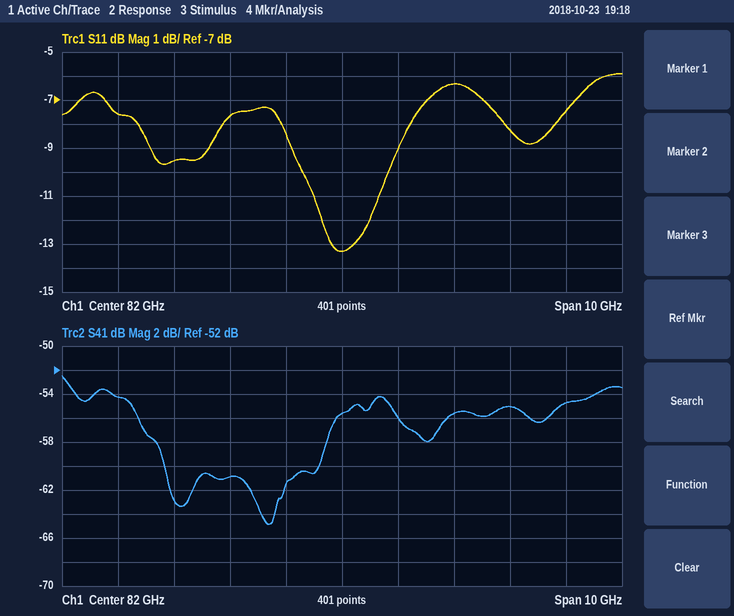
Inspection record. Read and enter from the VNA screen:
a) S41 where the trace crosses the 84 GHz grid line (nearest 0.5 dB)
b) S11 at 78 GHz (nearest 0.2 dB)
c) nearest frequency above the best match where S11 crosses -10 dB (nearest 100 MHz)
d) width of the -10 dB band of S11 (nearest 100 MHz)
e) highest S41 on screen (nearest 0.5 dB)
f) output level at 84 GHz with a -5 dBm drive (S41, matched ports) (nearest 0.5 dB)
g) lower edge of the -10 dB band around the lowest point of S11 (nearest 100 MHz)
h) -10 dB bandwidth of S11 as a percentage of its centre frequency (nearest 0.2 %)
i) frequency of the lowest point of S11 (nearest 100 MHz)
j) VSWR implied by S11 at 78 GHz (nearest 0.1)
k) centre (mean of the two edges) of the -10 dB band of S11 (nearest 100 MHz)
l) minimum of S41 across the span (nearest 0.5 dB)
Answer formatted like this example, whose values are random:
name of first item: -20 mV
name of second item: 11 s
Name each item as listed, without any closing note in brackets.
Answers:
S41 where the trace crosses the 84 GHz grid line: -55.5 dB
S11 at 78 GHz: -7.6 dB
nearest frequency above the best match where S11 crosses -10 dB: 82.8 GHz
width of the -10 dB band of S11: 1.5 GHz
highest S41 on screen: -52.5 dB
output level at 84 GHz with a -5 dBm drive (S41, matched ports): -60.5 dBm
lower edge of the -10 dB band around the lowest point of S11: 81.3 GHz
-10 dB bandwidth of S11 as a percentage of its centre frequency: 1.8 %
frequency of the lowest point of S11: 82.0 GHz
VSWR implied by S11 at 78 GHz: 2.4
centre (mean of the two edges) of the -10 dB band of S11: 82.1 GHz
minimum of S41 across the span: -65.0 dB
